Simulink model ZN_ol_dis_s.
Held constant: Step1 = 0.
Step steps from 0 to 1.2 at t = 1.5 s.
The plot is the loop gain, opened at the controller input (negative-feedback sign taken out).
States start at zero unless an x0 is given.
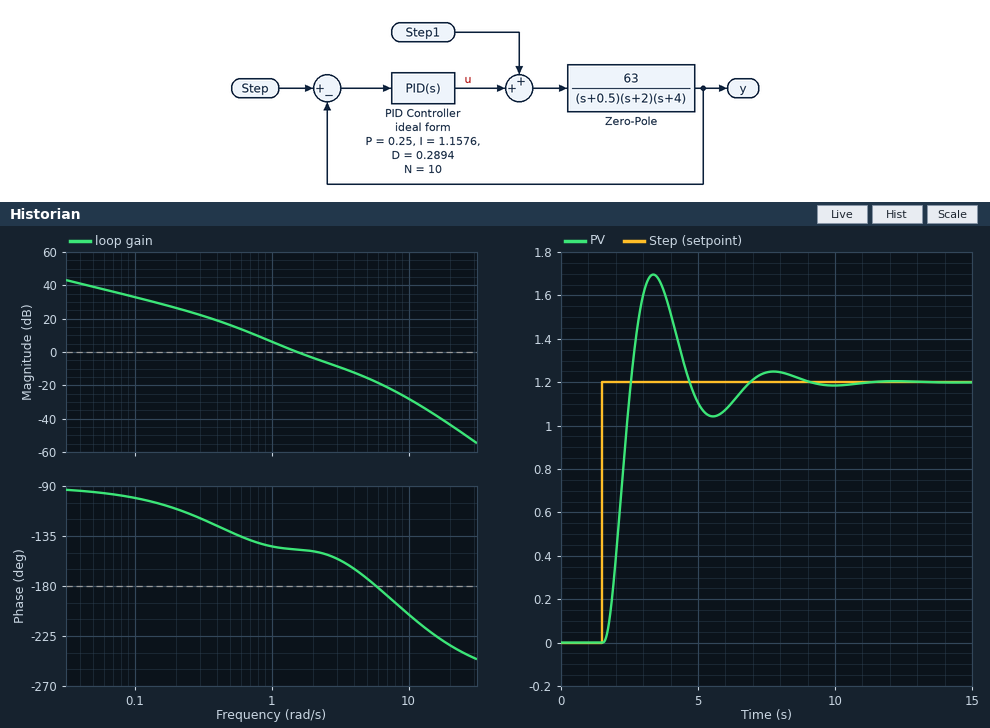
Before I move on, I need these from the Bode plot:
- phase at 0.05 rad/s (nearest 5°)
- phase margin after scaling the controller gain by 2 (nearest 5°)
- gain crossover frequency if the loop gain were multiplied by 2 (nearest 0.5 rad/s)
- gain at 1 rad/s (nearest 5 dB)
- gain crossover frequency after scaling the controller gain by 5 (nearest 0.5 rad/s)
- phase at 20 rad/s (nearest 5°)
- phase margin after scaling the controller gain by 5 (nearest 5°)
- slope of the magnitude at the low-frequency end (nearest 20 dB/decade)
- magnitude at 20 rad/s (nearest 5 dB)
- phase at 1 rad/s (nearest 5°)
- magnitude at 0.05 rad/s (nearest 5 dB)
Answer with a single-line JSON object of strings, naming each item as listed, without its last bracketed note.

{"phase at 0.05 rad/s": "-95°", "phase margin after scaling the controller gain by 2": "30°", "gain crossover frequency if the loop gain were multiplied by 2": "2.5 rad/s", "gain at 1 rad/s": "5 dB", "gain crossover frequency after scaling the controller gain by 5": "4.5 rad/s", "phase at 20 rad/s": "-235°", "phase margin after scaling the controller gain by 5": "10°", "slope of the magnitude at the low-frequency end": "-20 dB/decade", "magnitude at 20 rad/s": "-45 dB", "phase at 1 rad/s": "-145°", "magnitude at 0.05 rad/s": "40 dB"}
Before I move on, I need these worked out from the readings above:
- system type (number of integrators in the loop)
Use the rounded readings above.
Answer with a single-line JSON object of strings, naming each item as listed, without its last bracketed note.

{"system type": "1"}
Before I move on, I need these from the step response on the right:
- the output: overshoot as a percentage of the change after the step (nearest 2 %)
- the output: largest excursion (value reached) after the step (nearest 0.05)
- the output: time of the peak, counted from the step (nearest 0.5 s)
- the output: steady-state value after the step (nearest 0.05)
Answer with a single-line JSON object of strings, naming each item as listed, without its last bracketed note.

{"the output: overshoot as a percentage of the change after the step": "42 %", "the output: largest excursion (value reached) after the step": "1.70", "the output: time of the peak, counted from the step": "2.0 s", "the output: steady-state value after the step": "1.20"}
